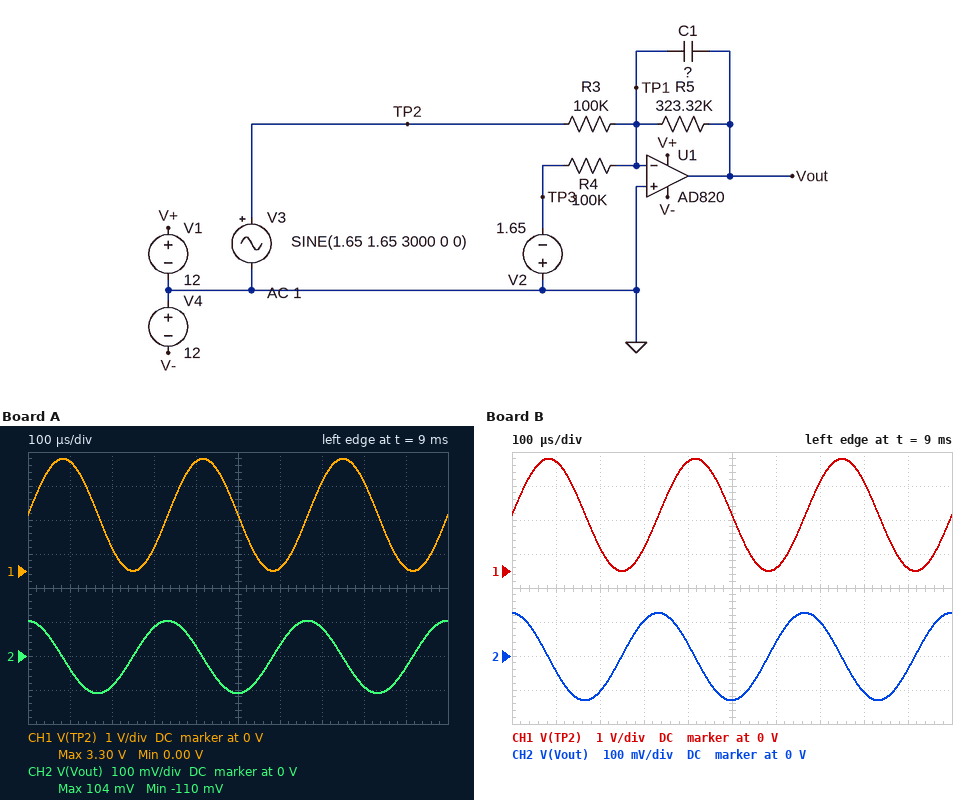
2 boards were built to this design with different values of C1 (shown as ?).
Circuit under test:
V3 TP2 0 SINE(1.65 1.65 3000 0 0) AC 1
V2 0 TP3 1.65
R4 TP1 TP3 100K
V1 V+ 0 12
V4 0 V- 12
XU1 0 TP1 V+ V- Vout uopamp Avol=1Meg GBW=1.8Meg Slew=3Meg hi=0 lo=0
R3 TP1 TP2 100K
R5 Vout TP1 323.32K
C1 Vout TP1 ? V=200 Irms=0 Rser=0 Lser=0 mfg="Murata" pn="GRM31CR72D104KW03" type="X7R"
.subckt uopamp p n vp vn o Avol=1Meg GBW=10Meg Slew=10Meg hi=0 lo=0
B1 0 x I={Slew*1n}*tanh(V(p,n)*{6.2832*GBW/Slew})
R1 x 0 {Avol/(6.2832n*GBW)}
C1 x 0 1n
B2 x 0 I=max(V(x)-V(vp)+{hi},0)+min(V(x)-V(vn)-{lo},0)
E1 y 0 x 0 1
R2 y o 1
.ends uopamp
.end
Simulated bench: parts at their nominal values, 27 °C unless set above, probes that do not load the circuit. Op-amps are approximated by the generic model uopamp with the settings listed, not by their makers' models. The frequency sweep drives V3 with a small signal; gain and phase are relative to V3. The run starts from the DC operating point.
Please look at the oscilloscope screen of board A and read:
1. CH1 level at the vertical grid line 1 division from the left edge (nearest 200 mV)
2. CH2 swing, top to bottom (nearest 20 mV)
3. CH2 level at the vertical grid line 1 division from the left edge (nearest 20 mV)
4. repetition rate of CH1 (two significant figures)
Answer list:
3.2 V
220 mV
-40 mV
3.0 kHz
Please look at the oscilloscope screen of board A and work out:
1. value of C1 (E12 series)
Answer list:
8.2 nF
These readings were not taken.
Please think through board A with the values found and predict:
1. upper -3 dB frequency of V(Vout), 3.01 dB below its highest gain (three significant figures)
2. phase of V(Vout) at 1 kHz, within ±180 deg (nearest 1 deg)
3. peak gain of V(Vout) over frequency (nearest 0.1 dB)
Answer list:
60.0 Hz
93 deg
10.2 dB
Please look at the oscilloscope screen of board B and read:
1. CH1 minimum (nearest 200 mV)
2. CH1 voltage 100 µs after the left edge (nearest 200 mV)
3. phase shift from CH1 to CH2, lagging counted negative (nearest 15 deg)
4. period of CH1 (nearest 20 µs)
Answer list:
0 V
3.2 V
90 deg
340 µs
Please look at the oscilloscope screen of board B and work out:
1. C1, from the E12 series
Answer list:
6.8 nF
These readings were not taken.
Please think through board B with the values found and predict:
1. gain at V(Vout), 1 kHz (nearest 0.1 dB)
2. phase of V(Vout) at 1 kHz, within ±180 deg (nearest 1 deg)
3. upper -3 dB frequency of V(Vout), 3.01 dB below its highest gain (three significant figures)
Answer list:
-12.6 dB
94 deg
72.4 Hz
